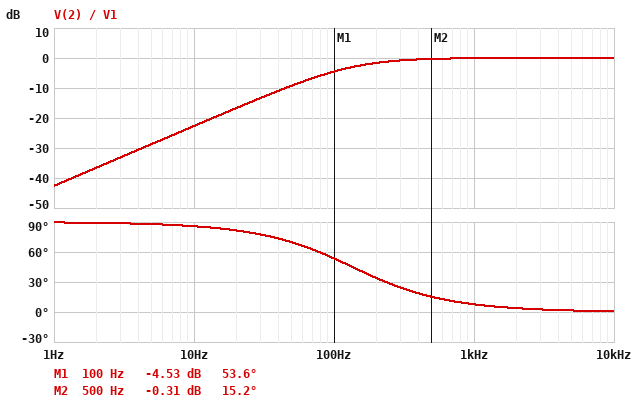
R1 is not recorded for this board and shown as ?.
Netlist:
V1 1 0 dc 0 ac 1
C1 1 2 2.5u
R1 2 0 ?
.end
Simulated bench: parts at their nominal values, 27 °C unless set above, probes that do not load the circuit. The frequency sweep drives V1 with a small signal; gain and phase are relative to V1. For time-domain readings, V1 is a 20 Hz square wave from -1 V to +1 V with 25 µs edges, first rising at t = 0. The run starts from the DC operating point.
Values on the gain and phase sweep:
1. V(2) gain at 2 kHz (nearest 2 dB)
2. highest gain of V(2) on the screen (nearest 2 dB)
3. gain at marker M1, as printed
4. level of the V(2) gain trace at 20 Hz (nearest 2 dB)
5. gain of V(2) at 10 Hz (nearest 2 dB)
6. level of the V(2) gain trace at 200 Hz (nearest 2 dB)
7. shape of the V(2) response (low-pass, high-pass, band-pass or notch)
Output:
0 dB
0 dB
-4.53 dB
-16 dB
-22 dB
-2 dB
high-pass
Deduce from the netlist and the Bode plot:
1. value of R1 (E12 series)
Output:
470 Ω
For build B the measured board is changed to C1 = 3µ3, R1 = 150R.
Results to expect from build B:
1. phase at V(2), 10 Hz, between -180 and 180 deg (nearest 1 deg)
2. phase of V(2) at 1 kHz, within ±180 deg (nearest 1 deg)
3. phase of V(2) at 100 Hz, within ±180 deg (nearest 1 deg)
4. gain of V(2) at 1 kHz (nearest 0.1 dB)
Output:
88 deg
18 deg
73 deg
-0.4 dB
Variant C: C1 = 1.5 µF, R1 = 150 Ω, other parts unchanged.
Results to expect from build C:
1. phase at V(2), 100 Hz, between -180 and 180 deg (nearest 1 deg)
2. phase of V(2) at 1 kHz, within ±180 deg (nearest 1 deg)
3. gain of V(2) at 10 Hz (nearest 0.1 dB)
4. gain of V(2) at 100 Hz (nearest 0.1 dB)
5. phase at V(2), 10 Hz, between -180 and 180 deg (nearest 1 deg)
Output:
82 deg
35 deg
-37.0 dB
-17.1 dB
89 deg
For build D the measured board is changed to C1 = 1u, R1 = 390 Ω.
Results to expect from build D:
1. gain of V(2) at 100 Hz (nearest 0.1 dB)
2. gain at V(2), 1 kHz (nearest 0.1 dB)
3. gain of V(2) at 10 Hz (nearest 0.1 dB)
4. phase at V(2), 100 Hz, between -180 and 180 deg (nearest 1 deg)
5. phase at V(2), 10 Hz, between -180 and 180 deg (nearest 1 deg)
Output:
-12.5 dB
-0.7 dB
-32.2 dB
76 deg
89 deg
